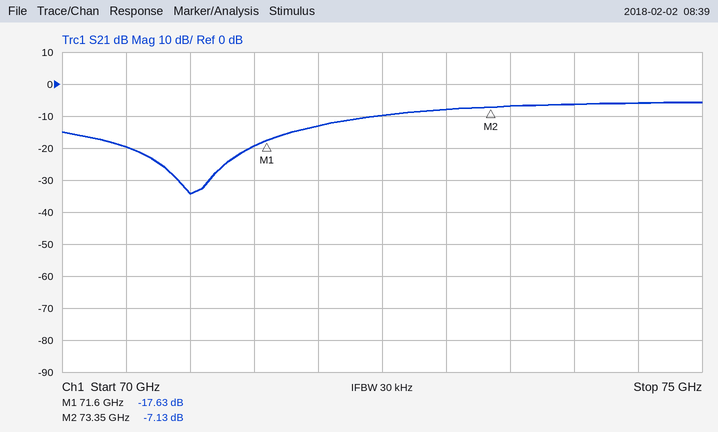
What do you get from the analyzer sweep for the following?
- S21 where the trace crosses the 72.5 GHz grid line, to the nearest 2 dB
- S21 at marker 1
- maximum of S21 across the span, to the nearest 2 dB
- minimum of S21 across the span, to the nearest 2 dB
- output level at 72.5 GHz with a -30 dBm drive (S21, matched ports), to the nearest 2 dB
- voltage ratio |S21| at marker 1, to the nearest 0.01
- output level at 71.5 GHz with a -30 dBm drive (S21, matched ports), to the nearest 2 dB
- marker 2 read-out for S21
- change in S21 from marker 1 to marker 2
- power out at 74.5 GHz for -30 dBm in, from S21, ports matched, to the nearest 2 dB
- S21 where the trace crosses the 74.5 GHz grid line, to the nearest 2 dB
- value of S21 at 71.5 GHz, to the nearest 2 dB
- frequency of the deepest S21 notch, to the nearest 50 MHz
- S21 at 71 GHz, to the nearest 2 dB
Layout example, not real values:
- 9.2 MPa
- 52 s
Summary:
- -10 dB
- -17.63 dB
- -6 dB
- -34 dB
- -40 dBm
- 0.13
- -50 dBm
- -7.13 dB
- 10.50 dB
- -36 dBm
- -6 dB
- -20 dB
- 71.00 GHz
- -34 dB
